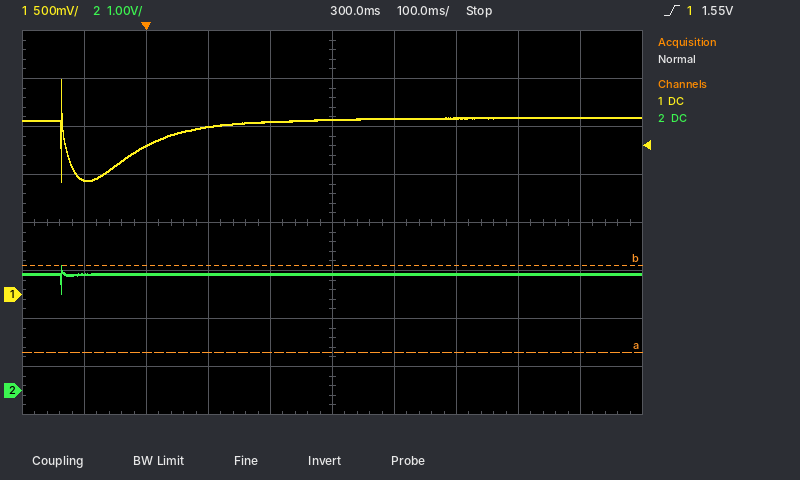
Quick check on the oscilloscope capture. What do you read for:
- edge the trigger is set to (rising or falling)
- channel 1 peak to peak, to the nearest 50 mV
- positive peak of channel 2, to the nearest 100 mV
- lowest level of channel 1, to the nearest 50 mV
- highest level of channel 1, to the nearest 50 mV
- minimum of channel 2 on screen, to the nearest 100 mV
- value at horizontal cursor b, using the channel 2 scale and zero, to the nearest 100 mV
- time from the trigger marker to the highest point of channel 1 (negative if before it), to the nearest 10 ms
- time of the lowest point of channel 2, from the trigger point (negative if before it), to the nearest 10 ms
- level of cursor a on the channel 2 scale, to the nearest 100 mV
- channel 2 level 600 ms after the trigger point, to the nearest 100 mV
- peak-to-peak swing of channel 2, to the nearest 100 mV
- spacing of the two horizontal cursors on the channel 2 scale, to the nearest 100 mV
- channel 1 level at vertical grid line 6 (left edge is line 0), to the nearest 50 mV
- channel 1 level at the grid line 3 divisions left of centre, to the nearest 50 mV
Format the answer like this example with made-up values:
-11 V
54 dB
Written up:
rising
1.05 V
2.6 V
1.20 V
2.25 V
2.0 V
2.6 V
-140 ms
-140 ms
800 mV
2.4 V
600 mV
1.8 V
1.85 V
1.55 V
